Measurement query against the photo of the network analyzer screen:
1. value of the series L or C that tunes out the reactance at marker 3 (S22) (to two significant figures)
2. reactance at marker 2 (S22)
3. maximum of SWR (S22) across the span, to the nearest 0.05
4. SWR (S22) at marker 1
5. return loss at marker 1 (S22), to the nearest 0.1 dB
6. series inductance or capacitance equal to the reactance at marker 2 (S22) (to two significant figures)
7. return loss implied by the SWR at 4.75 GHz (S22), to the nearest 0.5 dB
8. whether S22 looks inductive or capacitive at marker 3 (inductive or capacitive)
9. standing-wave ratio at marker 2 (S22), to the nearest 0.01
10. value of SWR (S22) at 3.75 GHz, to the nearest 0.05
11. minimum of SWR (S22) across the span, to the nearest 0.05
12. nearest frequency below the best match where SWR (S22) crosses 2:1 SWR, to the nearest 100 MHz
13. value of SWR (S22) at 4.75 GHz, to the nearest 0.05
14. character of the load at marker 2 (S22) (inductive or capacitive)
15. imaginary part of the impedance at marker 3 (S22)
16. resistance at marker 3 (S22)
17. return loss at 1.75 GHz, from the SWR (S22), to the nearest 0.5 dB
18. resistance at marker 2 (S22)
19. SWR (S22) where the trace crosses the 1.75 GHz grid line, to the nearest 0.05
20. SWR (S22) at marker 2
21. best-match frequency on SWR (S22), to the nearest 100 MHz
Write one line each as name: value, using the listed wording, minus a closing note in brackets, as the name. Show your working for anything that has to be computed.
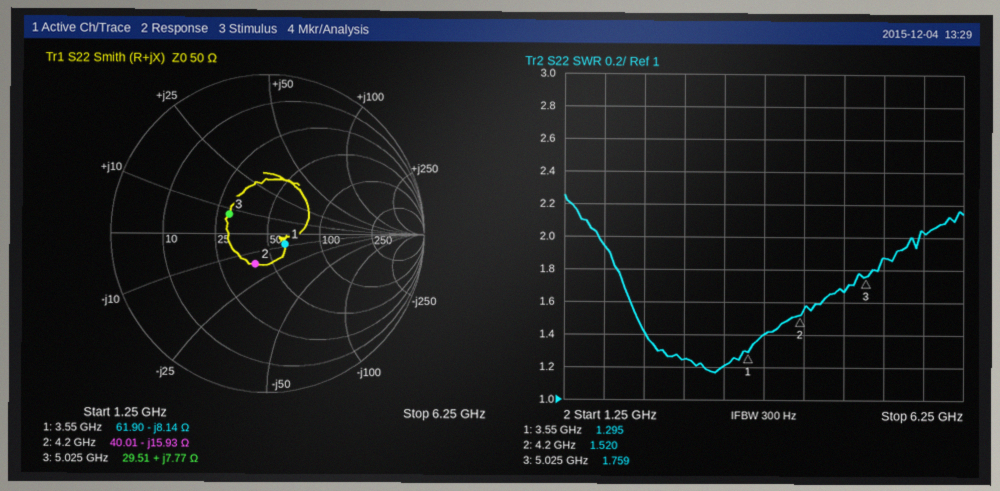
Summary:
value of the series L or C that tunes out the reactance at marker 3 (S22): C = 1/(2π × 5.025 GHz × 7.77 Ω) ≈ 4.1 pF
reactance at marker 2: -15.93 Ω
maximum of SWR (S22) across the span, to the nearest 0.05: 2.25
SWR (S22) at marker 1: 1.295
return loss at marker 1 (S22), to the nearest 0.1 dB: 17.8 dB
series inductance or capacitance equal to the reactance at marker 2 (S22): C = 1/(2π × 4.2 GHz × 15.93 Ω) ≈ 2.4 pF
return loss implied by the SWR at 4.75 GHz (S22), to the nearest 0.5 dB: −20 log10((1.65 − 1)/(1.65 + 1)) ≈ 12.2 dB, so 12.0 dB to the nearest 0.5 dB
whether S22 looks inductive or capacitive at marker 3: inductive
standing-wave ratio at marker 2 (S22), to the nearest 0.01: 1.52
value of SWR (S22) at 3.75 GHz, to the nearest 0.05: 1.40
minimum of SWR (S22) across the span, to the nearest 0.05: 1.15
nearest frequency below the best match where SWR (S22) crosses 2:1 SWR, to the nearest 100 MHz: 1.7 GHz
value of SWR (S22) at 4.75 GHz, to the nearest 0.05: 1.65
character of the load at marker 2 (S22): capacitive
imaginary part of the impedance at marker 3: +7.77 Ω
resistance at marker 3: 29.51 Ω
return loss at 1.75 GHz, from the SWR (S22), to the nearest 0.5 dB: −20 log10((1.95 − 1)/(1.95 + 1)) ≈ 9.84 dB, so 10.0 dB to the nearest 0.5 dB
resistance at marker 2: 40.01 Ω
SWR (S22) where the trace crosses the 1.75 GHz grid line, to the nearest 0.05: 1.95
SWR (S22) at marker 2: 1.520
best-match frequency on SWR (S22), to the nearest 100 MHz: 3.1 GHz
